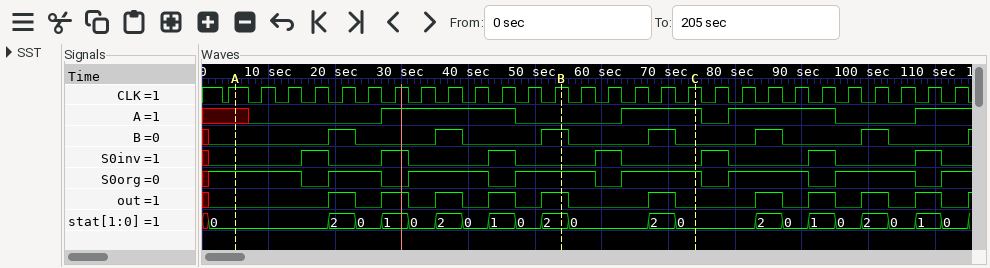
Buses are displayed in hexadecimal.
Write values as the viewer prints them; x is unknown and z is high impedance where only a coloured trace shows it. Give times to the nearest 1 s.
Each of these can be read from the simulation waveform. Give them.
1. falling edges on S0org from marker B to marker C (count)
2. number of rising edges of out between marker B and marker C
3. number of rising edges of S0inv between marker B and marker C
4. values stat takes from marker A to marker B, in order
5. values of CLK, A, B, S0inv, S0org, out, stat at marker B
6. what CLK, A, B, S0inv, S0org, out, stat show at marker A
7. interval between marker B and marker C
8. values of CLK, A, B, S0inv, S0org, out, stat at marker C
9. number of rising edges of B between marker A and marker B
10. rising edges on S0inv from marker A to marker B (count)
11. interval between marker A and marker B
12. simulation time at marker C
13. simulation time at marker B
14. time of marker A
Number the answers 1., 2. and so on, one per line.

1. 1
2. 1
3. 1
4. 0, 2, 0, 1, 0, 2, 0, 1, 0, 2
5. CLK=1, A=0, B=1, S0inv=0, S0org=1, out=1, stat=2
6. CLK=1, A=x, B=0, S0inv=0, S0org=1, out=0, stat=0
7. 20 s
8. CLK=1, A=1, B=0, S0inv=0, S0org=1, out=0, stat=0
9. 3
10. 3
11. 49 s
12. 74 s
13. 54 s
14. 5 s
